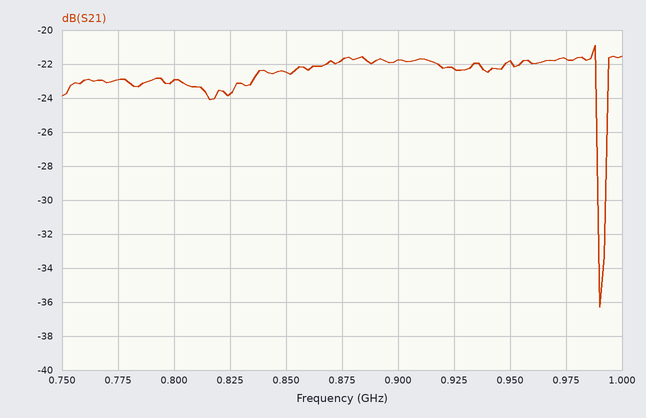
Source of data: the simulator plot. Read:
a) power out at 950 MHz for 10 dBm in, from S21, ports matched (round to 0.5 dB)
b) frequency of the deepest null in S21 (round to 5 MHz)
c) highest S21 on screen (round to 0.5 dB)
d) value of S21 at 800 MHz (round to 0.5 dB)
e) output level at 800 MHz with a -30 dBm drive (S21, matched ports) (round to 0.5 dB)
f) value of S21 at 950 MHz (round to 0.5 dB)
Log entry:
-12.0 dBm
990 MHz
-21.0 dB
-23.0 dB
-53.0 dBm
-22.0 dB
